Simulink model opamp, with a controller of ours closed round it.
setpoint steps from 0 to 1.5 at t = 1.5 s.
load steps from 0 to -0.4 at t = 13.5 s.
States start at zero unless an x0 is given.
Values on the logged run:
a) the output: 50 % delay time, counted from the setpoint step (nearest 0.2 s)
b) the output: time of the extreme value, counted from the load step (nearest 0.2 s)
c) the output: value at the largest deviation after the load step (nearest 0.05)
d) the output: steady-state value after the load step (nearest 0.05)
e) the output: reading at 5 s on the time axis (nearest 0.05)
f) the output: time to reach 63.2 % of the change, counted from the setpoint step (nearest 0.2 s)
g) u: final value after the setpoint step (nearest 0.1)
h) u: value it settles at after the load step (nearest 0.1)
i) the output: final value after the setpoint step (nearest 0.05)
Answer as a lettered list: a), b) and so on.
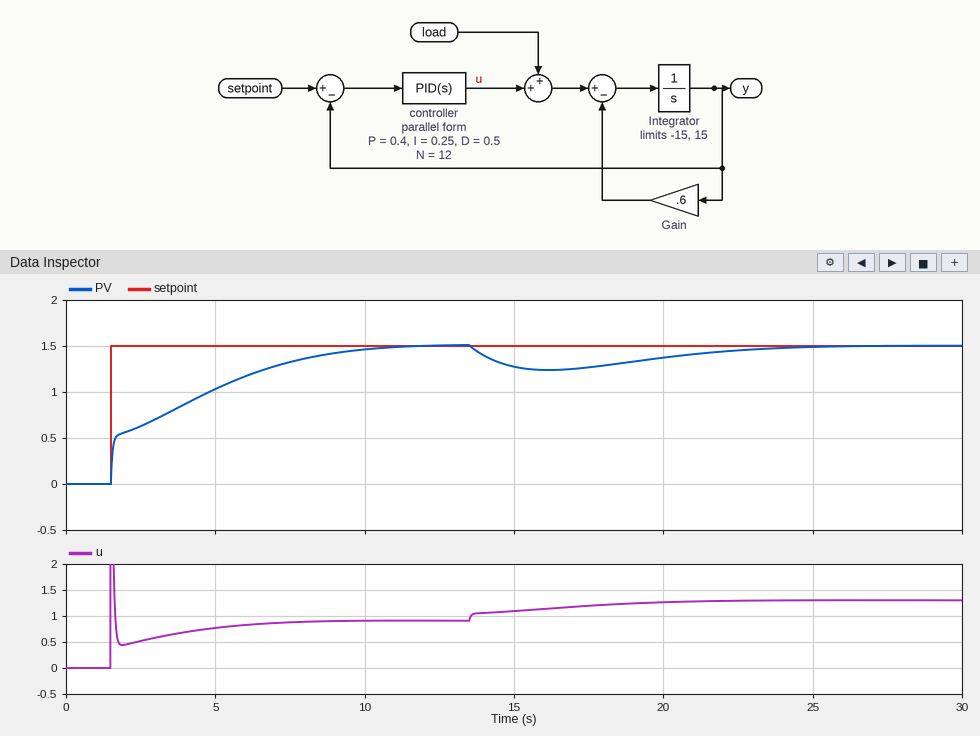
a) 1.8 s
b) 2.6 s
c) 1.25
d) 1.50
e) 1.05
f) 3.0 s
g) 0.9
h) 1.3
i) 1.50
